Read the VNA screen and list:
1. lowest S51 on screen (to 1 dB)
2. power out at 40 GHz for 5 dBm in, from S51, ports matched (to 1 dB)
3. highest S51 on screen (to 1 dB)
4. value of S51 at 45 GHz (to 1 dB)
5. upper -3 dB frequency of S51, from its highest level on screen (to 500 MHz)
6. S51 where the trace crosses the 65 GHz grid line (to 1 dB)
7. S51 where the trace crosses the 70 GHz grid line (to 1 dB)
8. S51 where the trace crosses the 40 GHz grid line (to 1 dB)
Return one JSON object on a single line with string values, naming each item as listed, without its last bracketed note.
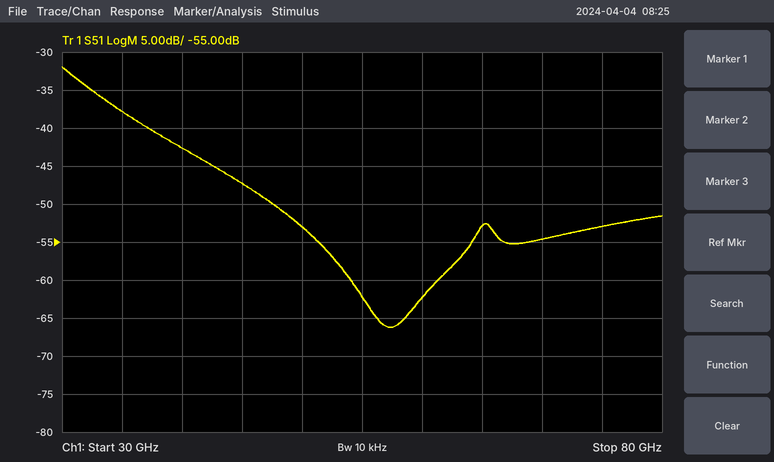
{"lowest S51 on screen": "-66 dB", "power out at 40 GHz for 5 dBm in, from S51, ports matched": "-38 dBm", "highest S51 on screen": "-32 dB", "value of S51 at 45 GHz": "-47 dB", "upper -3 dB frequency of S51, from its highest level on screen": "32.5 GHz", "S51 where the trace crosses the 65 GHz grid line": "-53 dB", "S51 where the trace crosses the 70 GHz grid line": "-55 dB", "S51 where the trace crosses the 40 GHz grid line": "-43 dB"}
